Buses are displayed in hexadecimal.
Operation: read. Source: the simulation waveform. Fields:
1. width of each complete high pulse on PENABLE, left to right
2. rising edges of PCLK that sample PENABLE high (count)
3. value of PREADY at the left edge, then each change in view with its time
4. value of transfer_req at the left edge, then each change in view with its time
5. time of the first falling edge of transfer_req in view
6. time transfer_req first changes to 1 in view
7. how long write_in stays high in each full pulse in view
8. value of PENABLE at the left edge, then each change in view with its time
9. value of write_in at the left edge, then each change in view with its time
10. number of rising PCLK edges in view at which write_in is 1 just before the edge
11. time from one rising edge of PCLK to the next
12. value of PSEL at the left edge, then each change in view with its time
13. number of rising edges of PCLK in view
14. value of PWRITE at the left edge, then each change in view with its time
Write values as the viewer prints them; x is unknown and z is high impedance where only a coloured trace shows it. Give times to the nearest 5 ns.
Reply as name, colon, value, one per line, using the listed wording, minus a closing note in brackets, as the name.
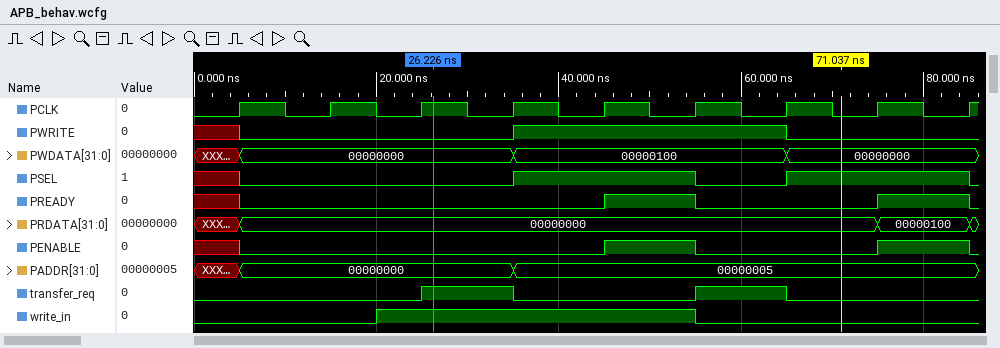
width of each complete high pulse on PENABLE, left to right: 10 ns, 10 ns
rising edges of PCLK that sample PENABLE high: 2
value of PREADY at the left edge, then each change in view with its time: x, 0 at 5 ns, 1 at 45 ns, 0 at 55 ns, 1 at 75 ns, 0 at 85 ns
value of transfer_req at the left edge, then each change in view with its time: 0, 1 at 25 ns, 0 at 35 ns, 1 at 55 ns, 0 at 65 ns
time of the first falling edge of transfer_req in view: 35 ns
time transfer_req first changes to 1 in view: 25 ns
how long write_in stays high in each full pulse in view: 35 ns
value of PENABLE at the left edge, then each change in view with its time: x, 0 at 5 ns, 1 at 45 ns, 0 at 55 ns, 1 at 75 ns, 0 at 85 ns
value of write_in at the left edge, then each change in view with its time: 0, 1 at 20 ns, 0 at 55 ns
number of rising PCLK edges in view at which write_in is 1 just before the edge: 4
time from one rising edge of PCLK to the next: 10 ns
value of PSEL at the left edge, then each change in view with its time: x, 0 at 5 ns, 1 at 35 ns, 0 at 55 ns, 1 at 65 ns, 0 at 85 ns
number of rising edges of PCLK in view: 9
value of PWRITE at the left edge, then each change in view with its time: x, 0 at 5 ns, 1 at 35 ns, 0 at 65 ns
